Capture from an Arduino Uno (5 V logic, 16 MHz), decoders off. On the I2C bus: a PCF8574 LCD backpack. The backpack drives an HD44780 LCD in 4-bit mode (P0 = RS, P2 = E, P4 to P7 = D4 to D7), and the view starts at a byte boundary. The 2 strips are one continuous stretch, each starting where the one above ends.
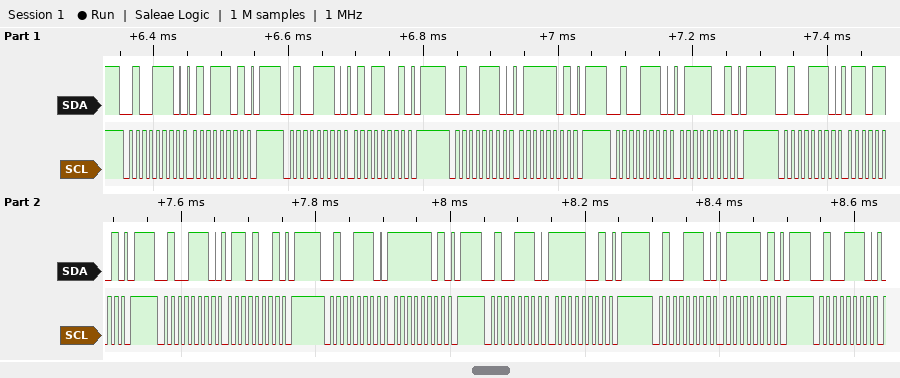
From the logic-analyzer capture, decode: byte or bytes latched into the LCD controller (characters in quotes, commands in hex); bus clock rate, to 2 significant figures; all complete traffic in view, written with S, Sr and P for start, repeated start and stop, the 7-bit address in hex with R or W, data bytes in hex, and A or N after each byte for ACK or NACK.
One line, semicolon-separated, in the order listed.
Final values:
'W' 'o'; 100 kHz; S 27W A 5D A P S 27W A 59 A P S 27W A 7D A P S 27W A 79 A P S 27W A 6D A P S 27W A 69 A P S 27W A FD A P S 27W A F9 A P S 27W A 7D A P S 27W A
